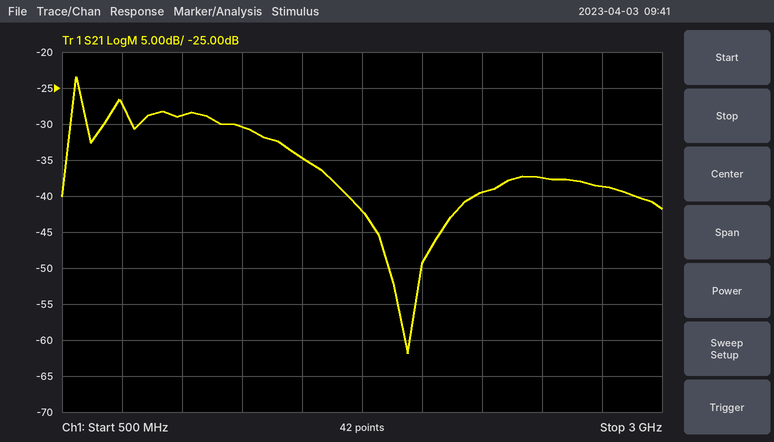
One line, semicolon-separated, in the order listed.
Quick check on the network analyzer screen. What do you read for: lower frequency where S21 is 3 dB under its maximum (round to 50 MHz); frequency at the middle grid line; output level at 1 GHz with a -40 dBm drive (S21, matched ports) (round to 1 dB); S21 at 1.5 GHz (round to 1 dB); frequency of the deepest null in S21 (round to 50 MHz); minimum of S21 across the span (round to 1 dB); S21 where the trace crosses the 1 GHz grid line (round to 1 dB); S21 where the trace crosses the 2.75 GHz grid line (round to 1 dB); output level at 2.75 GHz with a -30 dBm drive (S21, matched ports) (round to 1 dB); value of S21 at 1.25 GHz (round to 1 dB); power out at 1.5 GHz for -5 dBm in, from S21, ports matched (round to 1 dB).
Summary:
550 MHz; 1.75 GHz; -69 dBm; -35 dB; 1.95 GHz; -62 dB; -29 dB; -39 dB; -69 dBm; -30 dB; -40 dBm
